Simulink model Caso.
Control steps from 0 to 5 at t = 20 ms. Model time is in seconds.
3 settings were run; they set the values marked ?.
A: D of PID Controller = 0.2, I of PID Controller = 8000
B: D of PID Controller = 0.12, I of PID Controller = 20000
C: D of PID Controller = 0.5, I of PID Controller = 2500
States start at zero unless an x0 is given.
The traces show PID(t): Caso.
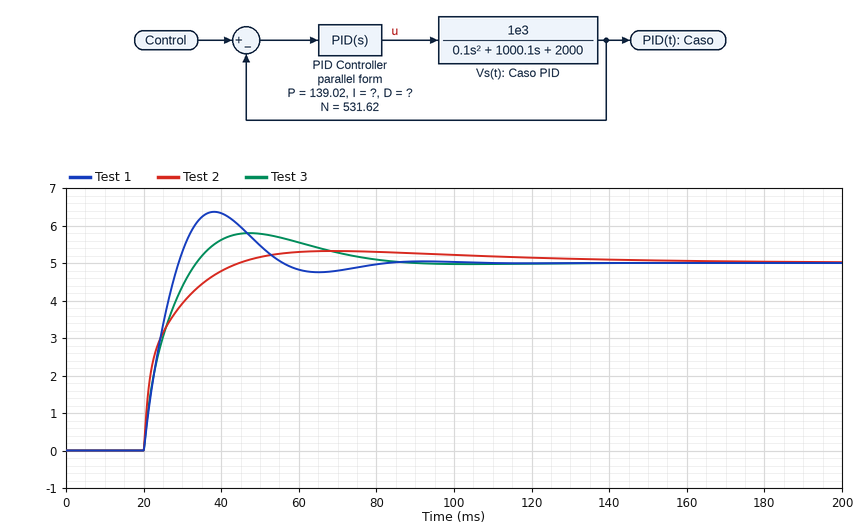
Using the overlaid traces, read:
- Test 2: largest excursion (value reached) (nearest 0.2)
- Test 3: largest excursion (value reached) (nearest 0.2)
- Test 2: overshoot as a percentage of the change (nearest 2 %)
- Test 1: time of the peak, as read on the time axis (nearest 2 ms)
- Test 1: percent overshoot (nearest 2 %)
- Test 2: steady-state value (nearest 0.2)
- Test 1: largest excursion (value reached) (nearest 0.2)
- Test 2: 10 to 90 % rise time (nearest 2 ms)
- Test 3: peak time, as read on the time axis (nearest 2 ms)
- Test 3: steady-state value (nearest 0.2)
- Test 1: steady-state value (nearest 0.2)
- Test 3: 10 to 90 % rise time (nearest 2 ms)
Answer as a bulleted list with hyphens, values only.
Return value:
- 5.4
- 5.8
- 6 %
- 38 ms
- 28 %
- 5.0
- 6.4
- 16 ms
- 48 ms
- 5.0
- 5.0
- 10 ms
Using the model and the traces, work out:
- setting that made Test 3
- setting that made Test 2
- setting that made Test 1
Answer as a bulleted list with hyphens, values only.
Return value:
- A
- C
- B
